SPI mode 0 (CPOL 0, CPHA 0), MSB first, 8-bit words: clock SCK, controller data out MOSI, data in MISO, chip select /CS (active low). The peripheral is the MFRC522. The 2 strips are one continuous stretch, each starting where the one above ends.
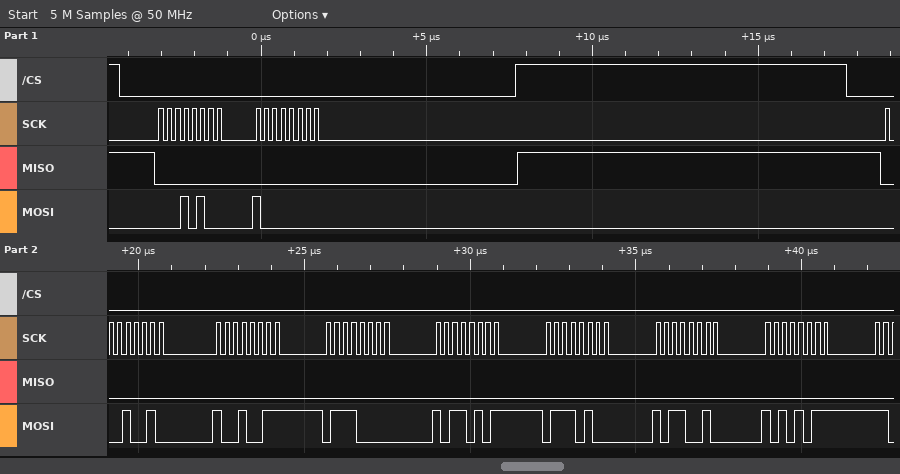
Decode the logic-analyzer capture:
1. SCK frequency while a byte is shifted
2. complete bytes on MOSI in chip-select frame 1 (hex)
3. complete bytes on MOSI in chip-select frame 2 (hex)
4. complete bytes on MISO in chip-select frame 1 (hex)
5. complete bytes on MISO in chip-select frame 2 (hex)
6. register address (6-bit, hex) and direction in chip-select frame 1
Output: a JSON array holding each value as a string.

["4 MHz", "14 80", "12 93 70 B5 74 B2 AB", "00 00", "00 00 00 00 00 00 00", "0x0A write"]
